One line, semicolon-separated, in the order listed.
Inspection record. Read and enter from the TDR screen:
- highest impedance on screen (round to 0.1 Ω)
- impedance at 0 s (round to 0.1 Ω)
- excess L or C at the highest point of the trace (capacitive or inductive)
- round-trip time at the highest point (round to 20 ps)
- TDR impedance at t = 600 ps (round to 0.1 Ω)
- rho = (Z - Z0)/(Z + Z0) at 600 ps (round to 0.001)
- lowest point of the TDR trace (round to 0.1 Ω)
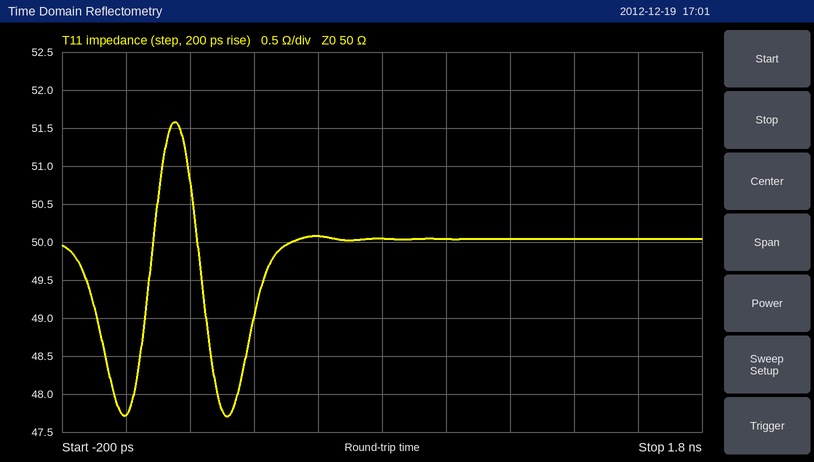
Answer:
51.6 Ω; 47.7 Ω; inductive; 160 ps; 50.1 Ω; +0.001; 47.7 Ω
